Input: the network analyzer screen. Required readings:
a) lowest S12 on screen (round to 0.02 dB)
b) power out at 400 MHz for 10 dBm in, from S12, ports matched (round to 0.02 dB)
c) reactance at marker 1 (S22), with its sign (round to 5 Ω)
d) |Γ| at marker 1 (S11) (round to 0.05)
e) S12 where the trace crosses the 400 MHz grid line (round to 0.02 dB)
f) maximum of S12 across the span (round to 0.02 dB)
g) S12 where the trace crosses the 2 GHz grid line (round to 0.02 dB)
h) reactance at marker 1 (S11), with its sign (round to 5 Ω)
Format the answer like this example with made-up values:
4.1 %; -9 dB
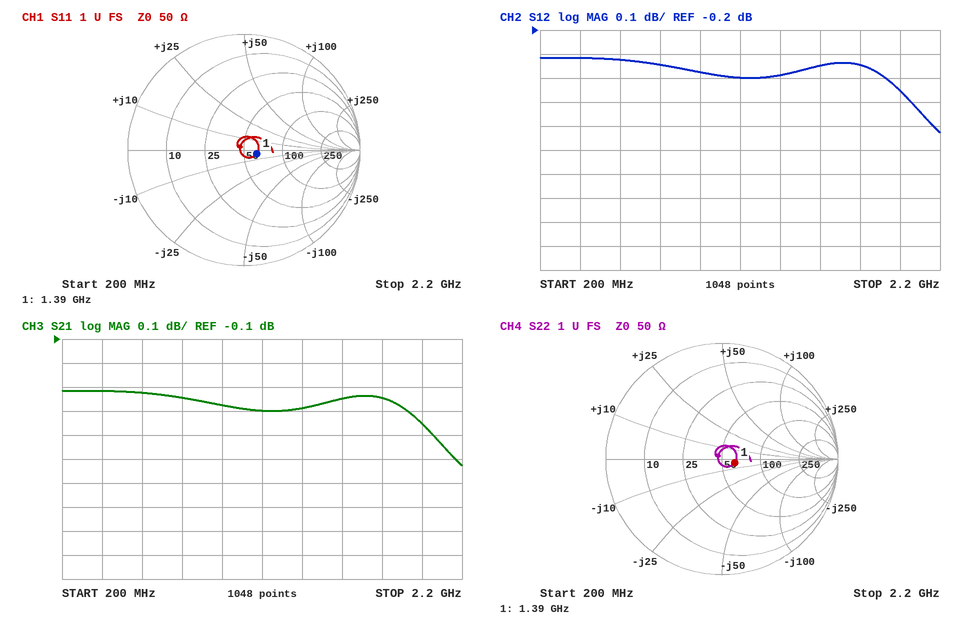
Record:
-0.62 dB; 9.68 dBm; -5 Ω; 0.10; -0.32 dB; -0.32 dB; -0.46 dB; -5 Ω
